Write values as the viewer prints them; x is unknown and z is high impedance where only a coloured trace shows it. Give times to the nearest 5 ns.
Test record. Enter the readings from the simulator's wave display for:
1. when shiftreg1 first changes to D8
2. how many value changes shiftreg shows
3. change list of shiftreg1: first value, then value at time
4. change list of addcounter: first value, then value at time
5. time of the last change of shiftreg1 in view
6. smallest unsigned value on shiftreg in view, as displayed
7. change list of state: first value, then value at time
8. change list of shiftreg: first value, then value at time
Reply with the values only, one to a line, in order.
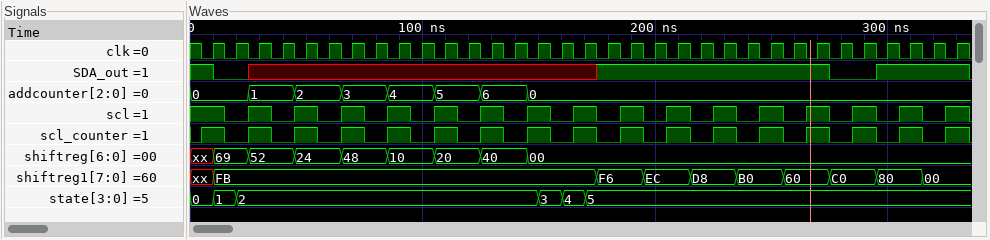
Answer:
215 ns
8
xx, FB at 10 ns, F6 at 175 ns, EC at 195 ns, D8 at 215 ns, B0 at 235 ns, 60 at 255 ns, C0 at 275 ns, 80 at 295 ns, 00 at 315 ns
0, 1 at 25 ns, 2 at 45 ns, 3 at 65 ns, 4 at 85 ns, 5 at 105 ns, 6 at 125 ns, 0 at 145 ns
315 ns
00
0, 1 at 10 ns, 2 at 20 ns, 3 at 150 ns, 4 at 160 ns, 5 at 170 ns
xx, 69 at 10 ns, 52 at 25 ns, 24 at 45 ns, 48 at 65 ns, 10 at 85 ns, 20 at 105 ns, 40 at 125 ns, 00 at 145 ns
